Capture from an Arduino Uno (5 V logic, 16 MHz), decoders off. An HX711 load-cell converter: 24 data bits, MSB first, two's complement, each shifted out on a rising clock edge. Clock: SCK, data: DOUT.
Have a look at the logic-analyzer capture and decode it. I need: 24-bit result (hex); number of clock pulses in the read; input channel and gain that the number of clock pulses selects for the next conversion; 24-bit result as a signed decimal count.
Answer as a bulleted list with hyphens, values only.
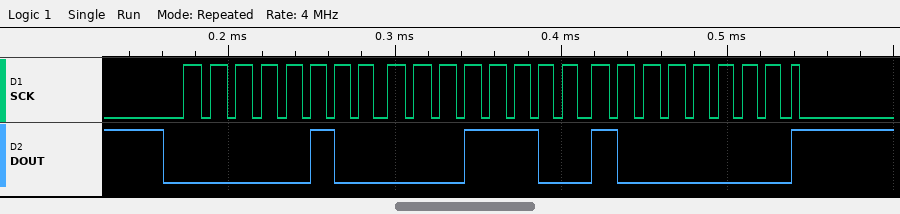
- 0x041C80
- 25
- channel A, gain 128
- 269440
